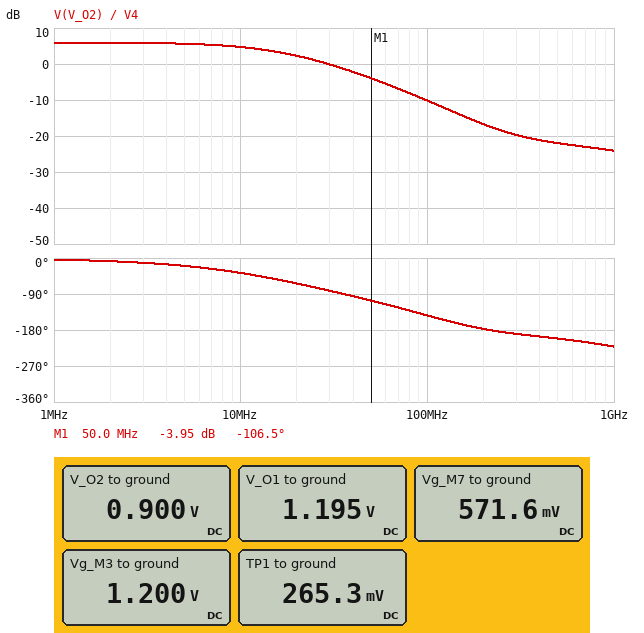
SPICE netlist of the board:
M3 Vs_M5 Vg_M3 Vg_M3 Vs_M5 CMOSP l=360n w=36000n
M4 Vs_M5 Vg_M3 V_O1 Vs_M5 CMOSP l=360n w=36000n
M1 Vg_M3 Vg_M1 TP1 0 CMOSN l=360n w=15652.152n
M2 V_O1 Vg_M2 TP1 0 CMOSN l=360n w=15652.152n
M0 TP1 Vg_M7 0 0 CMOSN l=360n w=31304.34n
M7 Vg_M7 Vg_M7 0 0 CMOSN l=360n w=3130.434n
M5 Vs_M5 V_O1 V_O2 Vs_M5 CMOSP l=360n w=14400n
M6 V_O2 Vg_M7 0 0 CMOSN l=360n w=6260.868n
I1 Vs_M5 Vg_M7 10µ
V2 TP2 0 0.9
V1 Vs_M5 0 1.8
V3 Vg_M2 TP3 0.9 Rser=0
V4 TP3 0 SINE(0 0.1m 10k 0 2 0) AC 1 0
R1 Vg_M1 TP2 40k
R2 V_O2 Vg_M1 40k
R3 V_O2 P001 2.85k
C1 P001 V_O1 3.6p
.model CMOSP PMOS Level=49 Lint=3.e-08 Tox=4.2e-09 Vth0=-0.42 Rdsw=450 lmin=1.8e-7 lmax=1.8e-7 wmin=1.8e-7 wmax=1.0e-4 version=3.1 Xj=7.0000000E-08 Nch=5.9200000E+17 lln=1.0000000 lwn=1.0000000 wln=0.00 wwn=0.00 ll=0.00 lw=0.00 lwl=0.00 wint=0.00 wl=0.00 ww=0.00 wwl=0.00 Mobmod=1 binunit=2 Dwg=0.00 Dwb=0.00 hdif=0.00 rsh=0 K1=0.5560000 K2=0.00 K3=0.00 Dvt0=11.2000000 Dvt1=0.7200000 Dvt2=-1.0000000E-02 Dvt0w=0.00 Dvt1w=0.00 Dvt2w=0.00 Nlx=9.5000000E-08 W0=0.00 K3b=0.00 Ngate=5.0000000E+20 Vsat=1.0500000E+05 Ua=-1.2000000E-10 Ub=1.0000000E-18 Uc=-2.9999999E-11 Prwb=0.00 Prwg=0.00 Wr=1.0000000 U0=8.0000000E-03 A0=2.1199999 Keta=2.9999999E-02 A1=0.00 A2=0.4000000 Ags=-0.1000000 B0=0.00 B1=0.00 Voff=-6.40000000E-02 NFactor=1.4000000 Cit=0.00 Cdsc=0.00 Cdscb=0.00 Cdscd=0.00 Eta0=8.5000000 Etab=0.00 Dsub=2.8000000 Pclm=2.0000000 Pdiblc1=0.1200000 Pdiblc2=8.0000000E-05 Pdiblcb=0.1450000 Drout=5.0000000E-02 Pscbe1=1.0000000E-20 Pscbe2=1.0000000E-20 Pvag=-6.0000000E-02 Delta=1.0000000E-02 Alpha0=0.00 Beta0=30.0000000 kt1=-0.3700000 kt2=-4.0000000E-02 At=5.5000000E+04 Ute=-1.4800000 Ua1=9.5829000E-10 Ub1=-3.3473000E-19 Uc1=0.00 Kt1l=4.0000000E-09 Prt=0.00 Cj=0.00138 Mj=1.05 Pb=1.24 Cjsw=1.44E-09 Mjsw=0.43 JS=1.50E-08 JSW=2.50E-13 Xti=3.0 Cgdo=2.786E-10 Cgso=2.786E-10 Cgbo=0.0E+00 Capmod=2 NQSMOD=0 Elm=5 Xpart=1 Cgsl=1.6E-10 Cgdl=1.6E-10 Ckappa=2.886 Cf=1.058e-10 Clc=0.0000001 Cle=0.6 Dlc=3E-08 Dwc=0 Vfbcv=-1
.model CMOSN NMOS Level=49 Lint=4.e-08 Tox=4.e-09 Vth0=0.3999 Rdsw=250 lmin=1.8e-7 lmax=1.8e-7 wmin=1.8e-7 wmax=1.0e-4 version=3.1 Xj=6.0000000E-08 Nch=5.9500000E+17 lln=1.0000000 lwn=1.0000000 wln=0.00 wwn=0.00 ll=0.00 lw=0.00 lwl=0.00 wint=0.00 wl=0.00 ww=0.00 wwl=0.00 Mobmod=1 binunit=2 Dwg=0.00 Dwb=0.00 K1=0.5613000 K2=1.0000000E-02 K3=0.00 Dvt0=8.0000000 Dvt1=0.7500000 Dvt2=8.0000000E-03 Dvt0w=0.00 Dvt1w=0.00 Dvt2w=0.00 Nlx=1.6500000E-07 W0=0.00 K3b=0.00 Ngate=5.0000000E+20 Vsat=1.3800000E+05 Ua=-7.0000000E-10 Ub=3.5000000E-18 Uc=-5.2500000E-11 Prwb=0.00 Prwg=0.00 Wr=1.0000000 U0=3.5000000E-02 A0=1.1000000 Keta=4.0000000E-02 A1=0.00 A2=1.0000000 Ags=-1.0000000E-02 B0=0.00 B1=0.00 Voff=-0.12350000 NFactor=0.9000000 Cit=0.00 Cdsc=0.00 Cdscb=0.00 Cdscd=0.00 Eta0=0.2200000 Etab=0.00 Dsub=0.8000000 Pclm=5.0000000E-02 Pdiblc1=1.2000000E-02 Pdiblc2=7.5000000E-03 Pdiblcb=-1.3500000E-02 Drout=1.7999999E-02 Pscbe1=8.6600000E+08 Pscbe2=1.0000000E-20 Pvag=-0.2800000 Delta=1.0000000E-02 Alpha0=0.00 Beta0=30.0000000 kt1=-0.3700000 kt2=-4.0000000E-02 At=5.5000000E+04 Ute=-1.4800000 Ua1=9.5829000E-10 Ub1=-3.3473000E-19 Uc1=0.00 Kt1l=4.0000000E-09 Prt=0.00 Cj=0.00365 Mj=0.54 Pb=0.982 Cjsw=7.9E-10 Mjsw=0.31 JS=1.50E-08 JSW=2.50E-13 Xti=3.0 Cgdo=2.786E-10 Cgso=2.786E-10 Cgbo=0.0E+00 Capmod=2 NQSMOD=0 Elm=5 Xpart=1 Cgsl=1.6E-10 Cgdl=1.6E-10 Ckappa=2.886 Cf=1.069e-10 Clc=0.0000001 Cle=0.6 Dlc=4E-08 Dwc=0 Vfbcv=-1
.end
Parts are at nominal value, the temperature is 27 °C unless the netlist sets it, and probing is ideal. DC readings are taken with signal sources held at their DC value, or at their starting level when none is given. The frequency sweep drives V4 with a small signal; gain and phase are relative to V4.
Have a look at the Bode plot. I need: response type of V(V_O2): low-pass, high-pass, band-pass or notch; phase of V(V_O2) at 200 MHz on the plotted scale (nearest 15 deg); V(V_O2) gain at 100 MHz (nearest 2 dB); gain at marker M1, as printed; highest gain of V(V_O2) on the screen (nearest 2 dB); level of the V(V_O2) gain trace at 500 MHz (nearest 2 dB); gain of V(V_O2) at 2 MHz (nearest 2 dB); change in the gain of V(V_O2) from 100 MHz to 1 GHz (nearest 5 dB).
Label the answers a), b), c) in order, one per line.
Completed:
a) low-pass
b) -180 deg
c) -10 dB
d) -3.95 dB
e) 6 dB
f) -22 dB
g) 6 dB
h) -15 dB
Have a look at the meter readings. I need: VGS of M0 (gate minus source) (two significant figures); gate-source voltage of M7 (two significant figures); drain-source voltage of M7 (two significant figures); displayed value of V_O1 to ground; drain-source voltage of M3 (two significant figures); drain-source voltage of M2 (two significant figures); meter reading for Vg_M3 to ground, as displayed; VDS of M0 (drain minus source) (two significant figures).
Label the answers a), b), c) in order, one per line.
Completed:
a) 570 mV
b) 570 mV
c) 570 mV
d) 1.195 V
e) 600 mV
f) 930 mV
g) 1.200 V
h) 270 mV
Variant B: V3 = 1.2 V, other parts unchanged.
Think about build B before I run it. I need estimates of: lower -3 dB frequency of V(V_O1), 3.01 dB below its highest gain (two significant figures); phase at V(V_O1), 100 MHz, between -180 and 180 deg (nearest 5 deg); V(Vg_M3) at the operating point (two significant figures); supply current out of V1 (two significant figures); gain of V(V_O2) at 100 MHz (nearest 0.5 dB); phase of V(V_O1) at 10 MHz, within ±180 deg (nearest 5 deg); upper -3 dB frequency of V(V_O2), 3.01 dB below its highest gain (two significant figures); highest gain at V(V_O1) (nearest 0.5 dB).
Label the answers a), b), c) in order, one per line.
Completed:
a) 13 MHz
b) 155 deg
c) 1.2 V
d) 140 µA
e) -9.5 dB
f) -135 deg
g) 15 MHz
h) 5.0 dB
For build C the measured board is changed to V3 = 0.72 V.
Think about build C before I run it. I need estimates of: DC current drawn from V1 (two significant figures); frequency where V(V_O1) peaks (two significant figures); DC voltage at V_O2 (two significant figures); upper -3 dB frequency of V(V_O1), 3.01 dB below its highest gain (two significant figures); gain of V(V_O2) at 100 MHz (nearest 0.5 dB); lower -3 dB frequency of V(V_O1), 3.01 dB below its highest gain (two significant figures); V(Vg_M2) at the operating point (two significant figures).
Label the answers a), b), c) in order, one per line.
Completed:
a) 110 µA
b) 40 MHz
c) 540 mV
d) 100 MHz
e) -4.5 dB
f) 16 MHz
g) 720 mV
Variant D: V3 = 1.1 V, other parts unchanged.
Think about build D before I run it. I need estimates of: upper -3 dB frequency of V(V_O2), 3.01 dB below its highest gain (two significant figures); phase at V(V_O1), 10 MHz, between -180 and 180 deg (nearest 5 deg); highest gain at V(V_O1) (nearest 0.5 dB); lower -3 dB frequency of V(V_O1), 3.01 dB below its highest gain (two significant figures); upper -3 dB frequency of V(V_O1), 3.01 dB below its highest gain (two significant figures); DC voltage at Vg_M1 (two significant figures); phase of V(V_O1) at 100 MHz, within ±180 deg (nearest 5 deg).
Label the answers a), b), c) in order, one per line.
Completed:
a) 15 MHz
b) -135 deg
c) 5.5 dB
d) 13 MHz
e) 190 MHz
f) 1.1 V
g) 155 deg
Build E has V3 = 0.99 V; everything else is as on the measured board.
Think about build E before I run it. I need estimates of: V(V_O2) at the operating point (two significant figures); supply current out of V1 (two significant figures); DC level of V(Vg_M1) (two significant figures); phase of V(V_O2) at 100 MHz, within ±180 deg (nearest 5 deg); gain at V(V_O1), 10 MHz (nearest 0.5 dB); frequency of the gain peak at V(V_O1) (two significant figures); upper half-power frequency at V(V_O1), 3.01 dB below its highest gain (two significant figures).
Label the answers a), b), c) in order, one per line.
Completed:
a) 1.1 V
b) 130 µA
c) 990 mV
d) -120 deg
e) 1.5 dB
f) 49 MHz
g) 170 MHz
